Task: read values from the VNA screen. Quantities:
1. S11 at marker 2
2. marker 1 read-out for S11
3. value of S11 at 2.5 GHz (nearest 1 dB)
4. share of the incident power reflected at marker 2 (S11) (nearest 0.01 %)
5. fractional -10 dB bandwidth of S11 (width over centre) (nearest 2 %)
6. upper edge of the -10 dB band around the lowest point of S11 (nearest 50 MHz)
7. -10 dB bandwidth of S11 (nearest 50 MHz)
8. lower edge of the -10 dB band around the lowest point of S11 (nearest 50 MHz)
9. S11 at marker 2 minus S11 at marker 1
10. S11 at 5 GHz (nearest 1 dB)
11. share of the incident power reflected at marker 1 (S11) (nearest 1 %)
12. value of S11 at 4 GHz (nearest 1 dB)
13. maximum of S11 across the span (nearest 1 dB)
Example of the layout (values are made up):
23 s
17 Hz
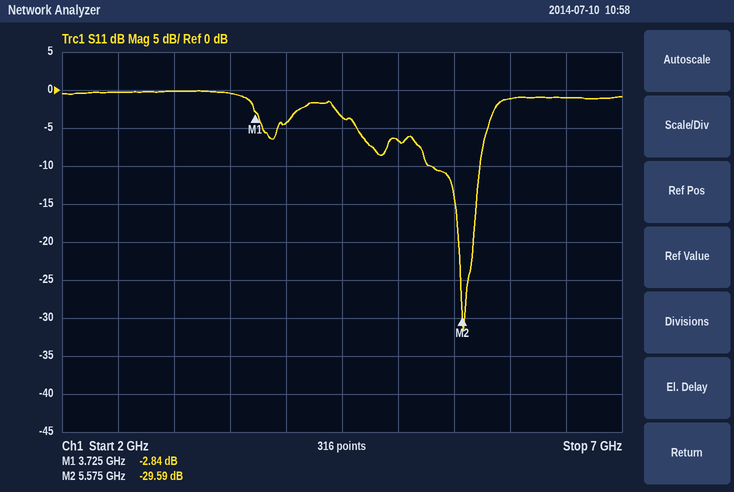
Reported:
-29.59 dB
-2.84 dB
0 dB
0.11 %
8 %
5.75 GHz
450 MHz
5.30 GHz
-26.75 dB
-7 dB
52 %
-4 dB
0 dB
